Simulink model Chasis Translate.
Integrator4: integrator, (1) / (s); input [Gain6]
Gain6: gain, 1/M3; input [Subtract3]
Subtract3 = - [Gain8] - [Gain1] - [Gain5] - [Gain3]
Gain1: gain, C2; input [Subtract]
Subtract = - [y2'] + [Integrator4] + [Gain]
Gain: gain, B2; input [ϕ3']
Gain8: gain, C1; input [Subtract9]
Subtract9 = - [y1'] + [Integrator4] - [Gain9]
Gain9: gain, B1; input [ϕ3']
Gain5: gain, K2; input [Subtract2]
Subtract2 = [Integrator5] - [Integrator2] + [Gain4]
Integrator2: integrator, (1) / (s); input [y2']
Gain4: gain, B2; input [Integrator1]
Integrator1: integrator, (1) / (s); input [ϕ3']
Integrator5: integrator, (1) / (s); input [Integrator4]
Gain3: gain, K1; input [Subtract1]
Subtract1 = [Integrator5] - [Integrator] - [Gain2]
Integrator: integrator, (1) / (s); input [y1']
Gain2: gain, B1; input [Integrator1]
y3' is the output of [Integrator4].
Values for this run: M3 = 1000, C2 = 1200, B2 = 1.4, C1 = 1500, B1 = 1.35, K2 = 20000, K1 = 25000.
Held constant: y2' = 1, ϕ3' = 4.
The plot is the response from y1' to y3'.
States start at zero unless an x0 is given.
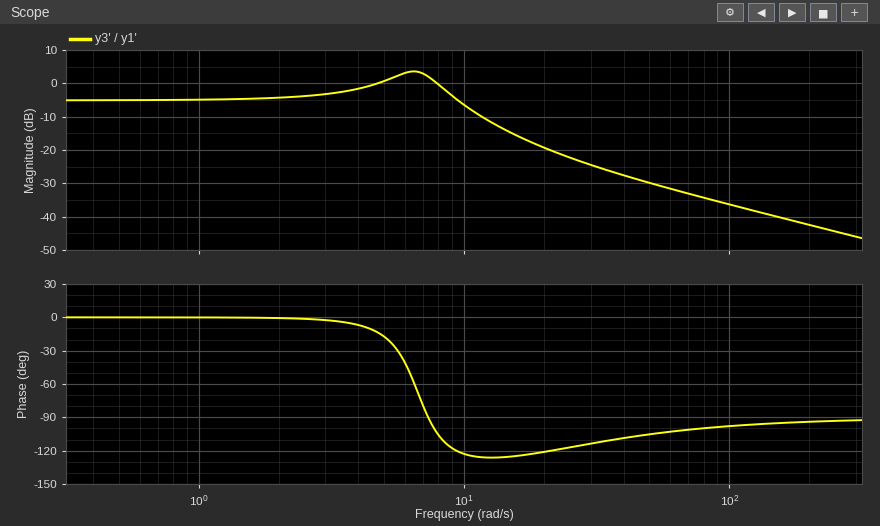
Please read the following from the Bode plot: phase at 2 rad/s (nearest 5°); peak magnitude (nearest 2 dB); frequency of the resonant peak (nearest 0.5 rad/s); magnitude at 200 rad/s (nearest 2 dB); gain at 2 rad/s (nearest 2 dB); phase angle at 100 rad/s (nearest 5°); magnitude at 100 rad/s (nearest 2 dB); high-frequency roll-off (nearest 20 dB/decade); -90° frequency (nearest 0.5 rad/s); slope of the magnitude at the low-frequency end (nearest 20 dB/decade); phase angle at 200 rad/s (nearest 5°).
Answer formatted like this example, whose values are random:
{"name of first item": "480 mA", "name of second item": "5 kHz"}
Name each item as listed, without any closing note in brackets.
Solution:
{"phase at 2 rad/s": "0°", "peak magnitude": "4 dB", "frequency of the resonant peak": "6.5 rad/s", "magnitude at 200 rad/s": "-42 dB", "gain at 2 rad/s": "-4 dB", "phase angle at 100 rad/s": "-100°", "magnitude at 100 rad/s": "-36 dB", "high-frequency roll-off": "-20 dB/decade", "-90° frequency": "7.5 rad/s", "slope of the magnitude at the low-frequency end": "0 dB/decade", "phase angle at 200 rad/s": "-95°"}
